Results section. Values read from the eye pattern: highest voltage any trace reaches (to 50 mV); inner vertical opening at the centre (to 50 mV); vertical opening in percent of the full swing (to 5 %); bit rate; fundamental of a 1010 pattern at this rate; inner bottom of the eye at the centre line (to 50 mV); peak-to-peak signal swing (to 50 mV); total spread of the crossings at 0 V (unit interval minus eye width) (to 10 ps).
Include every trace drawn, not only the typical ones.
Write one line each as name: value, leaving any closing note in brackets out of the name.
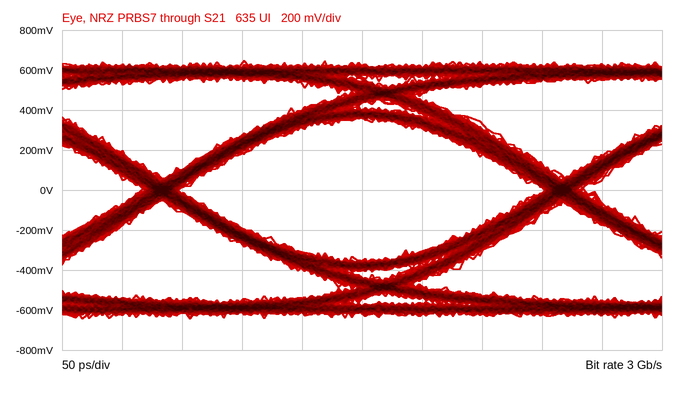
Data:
highest voltage any trace reaches: 650 mV
inner vertical opening at the centre: 700 mV
vertical opening in percent of the full swing: 55 %
bit rate: 3 Gb/s
fundamental of a 1010 pattern at this rate: 1.5 GHz
inner bottom of the eye at the centre line: -350 mV
peak-to-peak signal swing: 1.30 V
total spread of the crossings at 0 V (unit interval minus eye width): 30 ps
